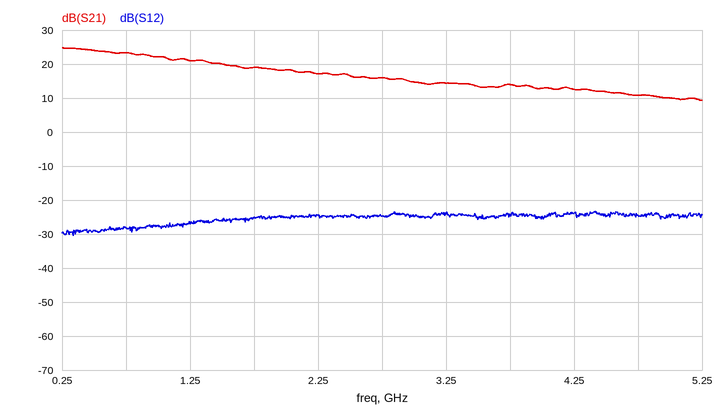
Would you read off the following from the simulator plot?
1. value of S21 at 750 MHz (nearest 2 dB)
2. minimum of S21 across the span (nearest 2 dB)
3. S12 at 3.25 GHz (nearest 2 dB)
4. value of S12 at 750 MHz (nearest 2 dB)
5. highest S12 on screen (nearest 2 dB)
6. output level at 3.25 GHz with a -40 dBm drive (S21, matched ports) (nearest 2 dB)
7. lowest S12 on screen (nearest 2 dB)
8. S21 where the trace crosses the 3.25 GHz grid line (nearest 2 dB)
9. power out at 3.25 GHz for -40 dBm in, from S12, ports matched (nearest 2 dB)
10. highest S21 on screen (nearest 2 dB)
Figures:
24 dB
10 dB
-24 dB
-28 dB
-24 dB
-26 dBm
-30 dB
14 dB
-64 dBm
24 dB
